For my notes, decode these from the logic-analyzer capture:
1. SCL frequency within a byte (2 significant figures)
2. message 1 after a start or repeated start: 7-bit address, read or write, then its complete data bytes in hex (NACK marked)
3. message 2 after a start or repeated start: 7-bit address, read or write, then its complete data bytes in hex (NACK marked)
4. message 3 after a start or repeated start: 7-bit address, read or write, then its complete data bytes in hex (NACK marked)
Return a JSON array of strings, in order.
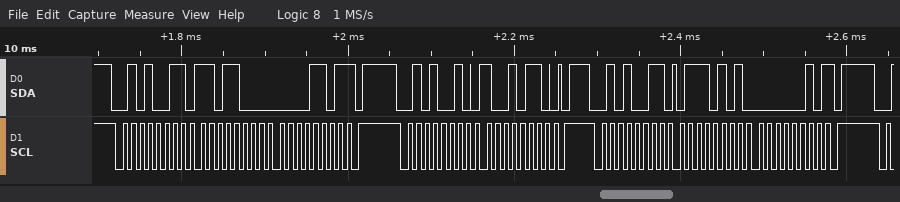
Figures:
["100 kHz", "0x29 read: D8 0D NACK", "0x29 write: 96", "0x29 read: 75 02 NACK"]
